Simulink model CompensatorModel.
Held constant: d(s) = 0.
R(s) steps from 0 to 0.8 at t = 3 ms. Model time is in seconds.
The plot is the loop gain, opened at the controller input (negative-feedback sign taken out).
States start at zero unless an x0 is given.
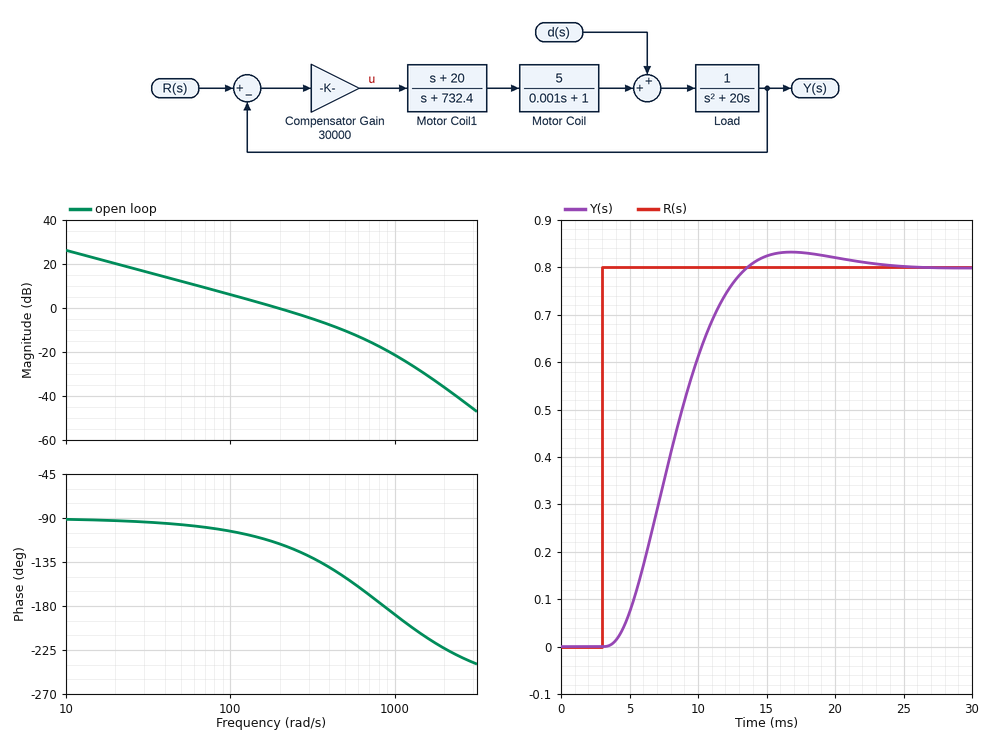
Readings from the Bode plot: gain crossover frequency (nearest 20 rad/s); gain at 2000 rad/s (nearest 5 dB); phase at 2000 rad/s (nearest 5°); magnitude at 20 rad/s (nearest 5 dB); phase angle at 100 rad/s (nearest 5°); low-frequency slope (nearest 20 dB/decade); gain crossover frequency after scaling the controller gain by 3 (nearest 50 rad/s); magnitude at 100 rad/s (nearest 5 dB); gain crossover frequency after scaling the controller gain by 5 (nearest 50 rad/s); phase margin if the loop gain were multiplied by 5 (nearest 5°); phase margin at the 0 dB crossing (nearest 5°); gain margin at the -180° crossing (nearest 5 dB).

200 rad/s
-35 dB
-225°
20 dB
-105°
-20 dB/decade
450 rad/s
5 dB
650 rad/s
15°
65°
20 dB
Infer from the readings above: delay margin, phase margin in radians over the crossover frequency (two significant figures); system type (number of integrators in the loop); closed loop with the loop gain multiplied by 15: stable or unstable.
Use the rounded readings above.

0.0057 s
1
unstable
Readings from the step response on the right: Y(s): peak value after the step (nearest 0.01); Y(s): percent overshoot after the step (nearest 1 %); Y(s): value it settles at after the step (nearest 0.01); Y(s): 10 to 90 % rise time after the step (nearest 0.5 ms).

0.83
4 %
0.80
6.5 ms
